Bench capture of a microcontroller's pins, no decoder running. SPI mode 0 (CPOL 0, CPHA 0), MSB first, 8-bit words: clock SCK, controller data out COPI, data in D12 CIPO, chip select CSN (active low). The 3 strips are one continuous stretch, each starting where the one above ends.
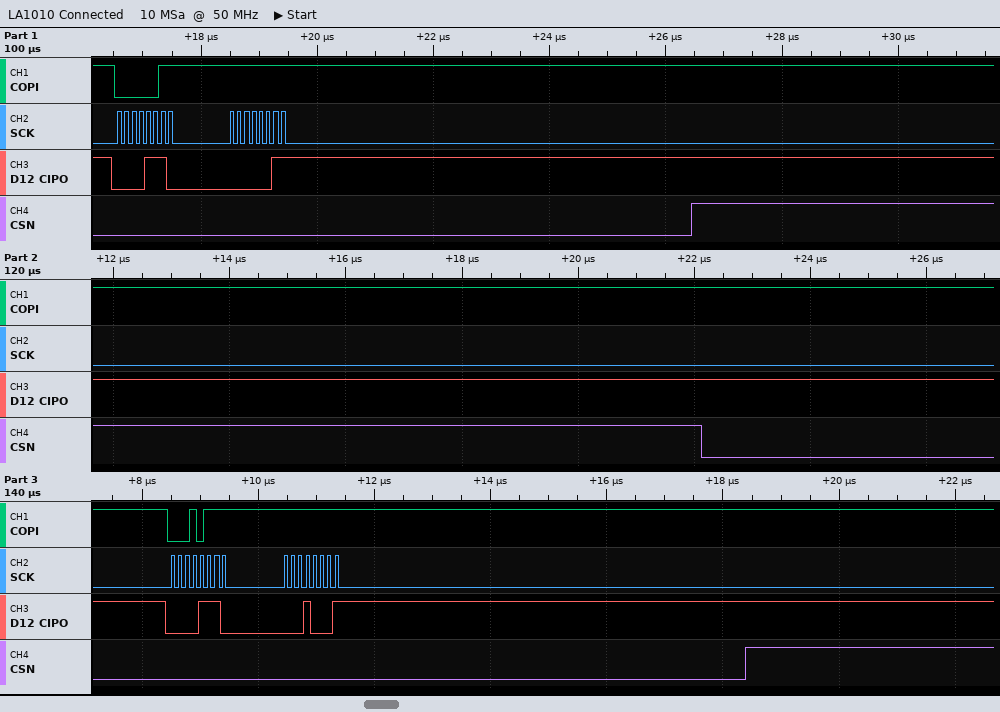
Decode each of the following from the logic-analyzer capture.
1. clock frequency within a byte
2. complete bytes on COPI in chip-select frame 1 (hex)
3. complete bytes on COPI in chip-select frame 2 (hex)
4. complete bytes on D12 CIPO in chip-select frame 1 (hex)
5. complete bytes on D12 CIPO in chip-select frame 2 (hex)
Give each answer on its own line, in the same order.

8 MHz
03 FF
17 FF
0E 03
0E 11
